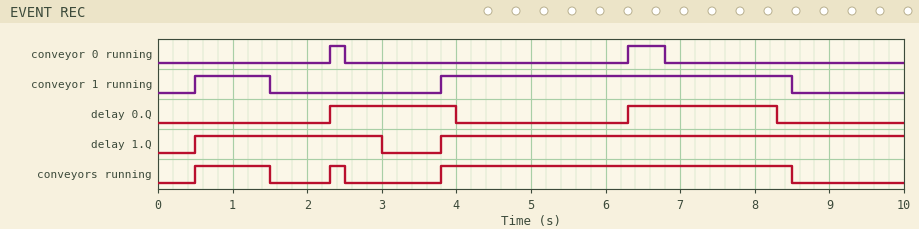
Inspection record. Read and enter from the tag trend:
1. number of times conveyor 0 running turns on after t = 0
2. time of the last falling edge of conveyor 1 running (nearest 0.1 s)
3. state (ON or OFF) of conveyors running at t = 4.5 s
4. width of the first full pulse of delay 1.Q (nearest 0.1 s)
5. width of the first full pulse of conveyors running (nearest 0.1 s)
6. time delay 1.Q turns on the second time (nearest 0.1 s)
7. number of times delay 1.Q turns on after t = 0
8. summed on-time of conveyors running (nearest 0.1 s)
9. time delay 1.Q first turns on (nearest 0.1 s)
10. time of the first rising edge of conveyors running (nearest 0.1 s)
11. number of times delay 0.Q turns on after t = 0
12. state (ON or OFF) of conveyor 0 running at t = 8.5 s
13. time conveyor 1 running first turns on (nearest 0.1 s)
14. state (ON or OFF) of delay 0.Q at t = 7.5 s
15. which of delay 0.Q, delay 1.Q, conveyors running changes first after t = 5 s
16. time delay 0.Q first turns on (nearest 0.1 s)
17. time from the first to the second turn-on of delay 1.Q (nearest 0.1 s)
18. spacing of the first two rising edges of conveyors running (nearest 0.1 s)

2
8.5 s
ON
2.5 s
1.0 s
3.8 s
2
5.9 s
0.5 s
0.5 s
2
OFF
0.5 s
ON
delay 0.Q
2.3 s
3.3 s
1.8 s
